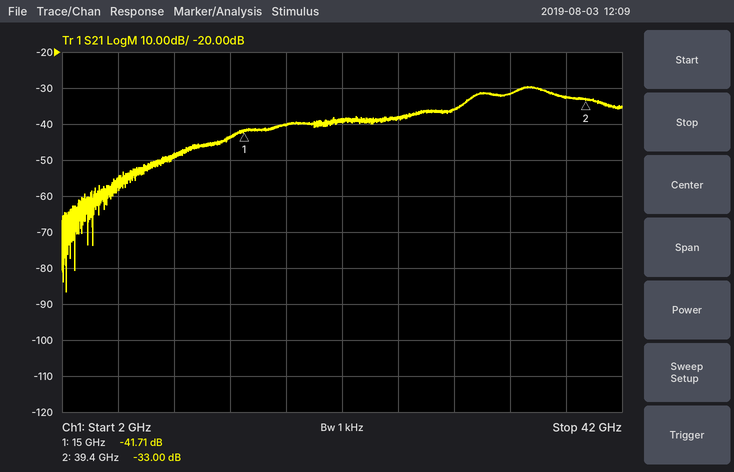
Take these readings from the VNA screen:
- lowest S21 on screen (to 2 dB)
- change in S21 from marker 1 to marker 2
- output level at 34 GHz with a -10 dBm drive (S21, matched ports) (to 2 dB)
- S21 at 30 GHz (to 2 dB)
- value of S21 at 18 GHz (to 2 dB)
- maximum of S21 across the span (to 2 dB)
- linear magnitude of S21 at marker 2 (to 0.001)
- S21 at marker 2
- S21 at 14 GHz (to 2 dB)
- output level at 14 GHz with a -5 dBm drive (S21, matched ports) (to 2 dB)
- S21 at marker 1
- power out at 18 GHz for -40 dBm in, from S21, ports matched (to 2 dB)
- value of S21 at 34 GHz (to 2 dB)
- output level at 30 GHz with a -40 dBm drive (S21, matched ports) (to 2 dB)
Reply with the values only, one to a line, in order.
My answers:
-86 dB
8.71 dB
-42 dBm
-36 dB
-40 dB
-30 dB
0.022
-33.00 dB
-44 dB
-48 dBm
-41.71 dB
-80 dBm
-32 dB
-76 dBm
